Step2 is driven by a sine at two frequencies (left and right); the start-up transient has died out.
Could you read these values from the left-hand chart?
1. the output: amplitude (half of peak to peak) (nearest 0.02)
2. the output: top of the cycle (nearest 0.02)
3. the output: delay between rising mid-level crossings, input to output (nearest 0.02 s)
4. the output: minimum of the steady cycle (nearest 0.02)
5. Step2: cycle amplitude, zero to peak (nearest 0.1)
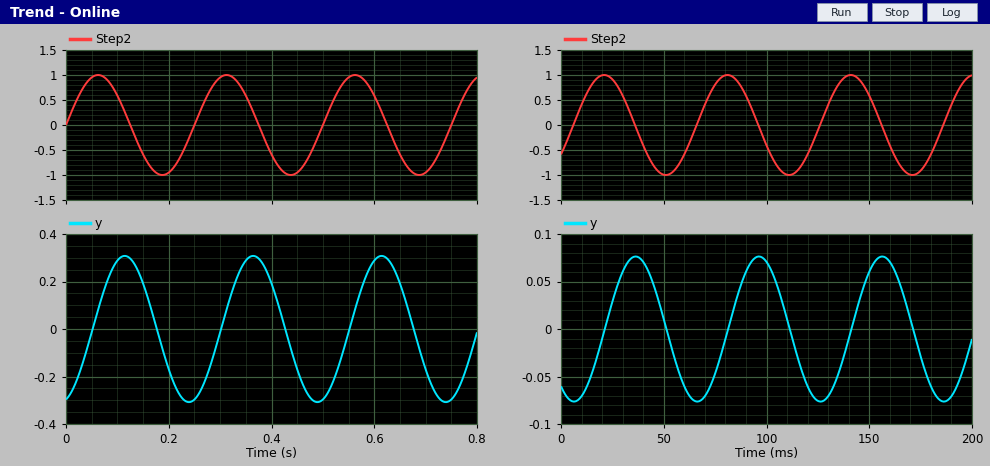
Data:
0.30
0.30
0.06 s
-0.30
1.0
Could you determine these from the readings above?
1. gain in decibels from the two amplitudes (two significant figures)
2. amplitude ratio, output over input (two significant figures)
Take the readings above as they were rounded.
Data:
-10 dB
0.30
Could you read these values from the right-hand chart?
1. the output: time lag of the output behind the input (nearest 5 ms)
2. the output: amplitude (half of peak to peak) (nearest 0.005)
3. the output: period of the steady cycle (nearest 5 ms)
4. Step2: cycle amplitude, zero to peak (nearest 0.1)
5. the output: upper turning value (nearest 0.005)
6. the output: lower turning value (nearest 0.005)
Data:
15 ms
0.075
60 ms
1.0
0.075
-0.075
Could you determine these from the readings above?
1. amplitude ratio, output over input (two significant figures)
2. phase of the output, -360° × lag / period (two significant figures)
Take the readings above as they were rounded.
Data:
0.075
-90°
